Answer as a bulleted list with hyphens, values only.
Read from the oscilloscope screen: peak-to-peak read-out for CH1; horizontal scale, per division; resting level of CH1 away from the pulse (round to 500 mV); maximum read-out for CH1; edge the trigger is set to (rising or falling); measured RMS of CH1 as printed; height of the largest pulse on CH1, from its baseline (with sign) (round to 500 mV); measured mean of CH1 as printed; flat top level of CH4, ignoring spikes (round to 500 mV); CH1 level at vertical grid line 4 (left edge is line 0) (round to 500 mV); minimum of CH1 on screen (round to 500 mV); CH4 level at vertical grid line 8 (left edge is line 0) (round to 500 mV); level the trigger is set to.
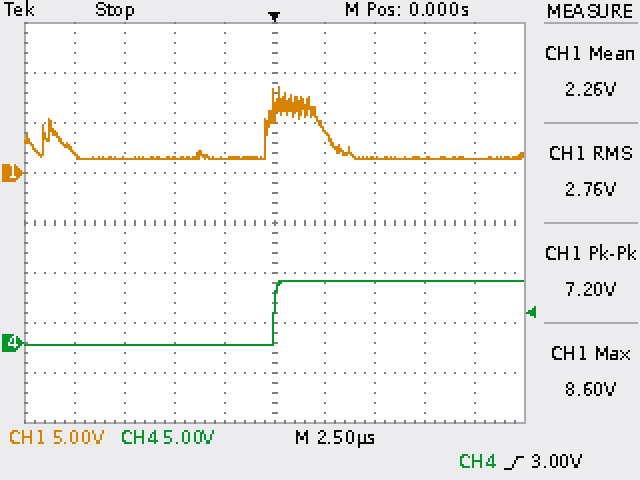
- 7.20 V
- 2.5 µs
- 1.5 V
- 8.60 V
- rising
- 2.76 V
- +7.0 V
- 2.26 V
- 6.0 V
- 1.5 V
- 1.5 V
- 6.0 V
- 3.00 V
